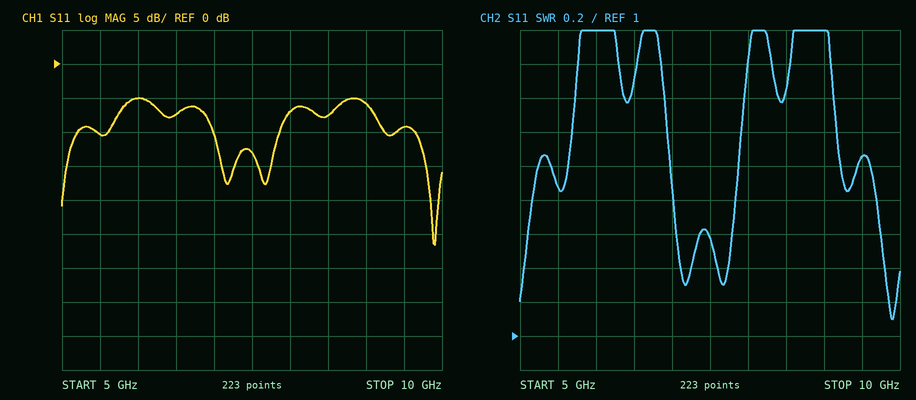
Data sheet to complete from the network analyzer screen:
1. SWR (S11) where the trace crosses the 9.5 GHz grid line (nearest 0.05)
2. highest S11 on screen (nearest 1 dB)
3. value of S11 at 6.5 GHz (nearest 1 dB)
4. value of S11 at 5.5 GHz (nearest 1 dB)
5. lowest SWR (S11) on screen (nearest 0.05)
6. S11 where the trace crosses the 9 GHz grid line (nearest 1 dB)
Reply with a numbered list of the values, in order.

1. 2.05
2. -5 dB
3. -7 dB
4. -10 dB
5. 1.10
6. -6 dB
